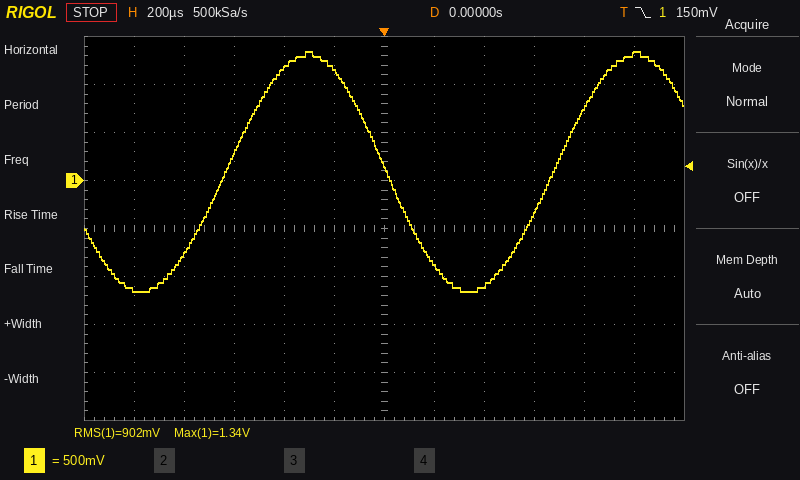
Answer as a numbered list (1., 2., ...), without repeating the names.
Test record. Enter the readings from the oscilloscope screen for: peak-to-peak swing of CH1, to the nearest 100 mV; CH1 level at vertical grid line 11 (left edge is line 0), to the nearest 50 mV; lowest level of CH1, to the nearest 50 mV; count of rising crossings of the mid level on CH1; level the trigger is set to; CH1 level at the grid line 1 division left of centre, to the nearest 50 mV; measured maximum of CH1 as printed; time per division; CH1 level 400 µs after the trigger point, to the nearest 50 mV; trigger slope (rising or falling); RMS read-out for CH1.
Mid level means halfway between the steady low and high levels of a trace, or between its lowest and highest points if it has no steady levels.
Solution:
1. 2.50 V
2. 1.30 V
3. -1.15 V
4. 2
5. 150 mV
6. 1.15 V
7. 1.34 V
8. 200 µs
9. -1.10 V
10. falling
11. 902 mV
